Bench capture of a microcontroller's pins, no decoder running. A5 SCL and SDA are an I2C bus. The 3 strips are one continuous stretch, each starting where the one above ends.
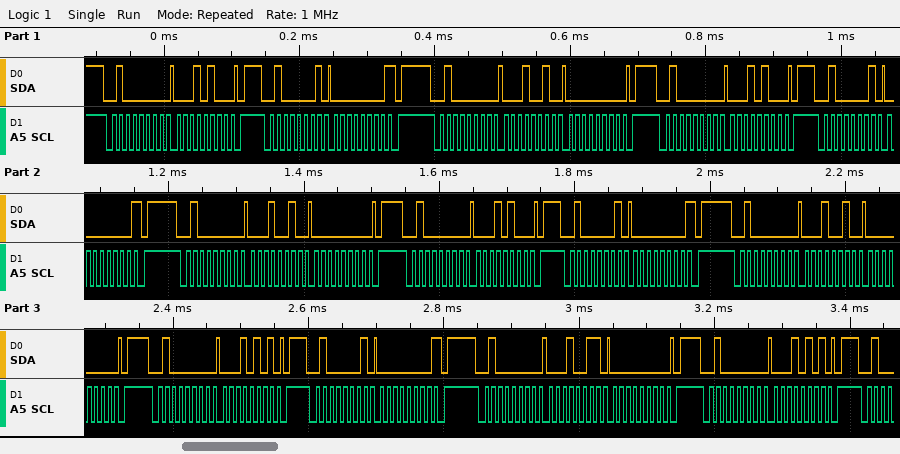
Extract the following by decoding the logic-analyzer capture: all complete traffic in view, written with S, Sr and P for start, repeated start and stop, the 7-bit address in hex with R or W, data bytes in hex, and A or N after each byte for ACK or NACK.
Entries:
S 20W A 14 A P S 20R A 00 N P S 20W A 12 A 00 A P S 20W A 14 A P S 20R A 00 N P S 20W A 12 A 00 A P S 20W A 14 A P S 20R A 00 N P S 20W A 12 A 00 A P S 20W A 15 A P S 20R A 00 N P S 20W A 13 A 00 A P S 20W A 15 A P
